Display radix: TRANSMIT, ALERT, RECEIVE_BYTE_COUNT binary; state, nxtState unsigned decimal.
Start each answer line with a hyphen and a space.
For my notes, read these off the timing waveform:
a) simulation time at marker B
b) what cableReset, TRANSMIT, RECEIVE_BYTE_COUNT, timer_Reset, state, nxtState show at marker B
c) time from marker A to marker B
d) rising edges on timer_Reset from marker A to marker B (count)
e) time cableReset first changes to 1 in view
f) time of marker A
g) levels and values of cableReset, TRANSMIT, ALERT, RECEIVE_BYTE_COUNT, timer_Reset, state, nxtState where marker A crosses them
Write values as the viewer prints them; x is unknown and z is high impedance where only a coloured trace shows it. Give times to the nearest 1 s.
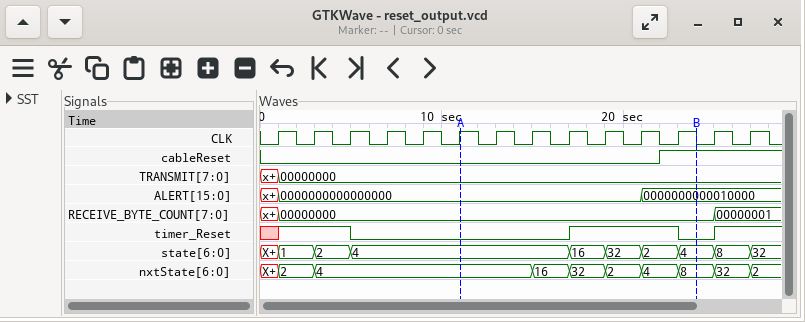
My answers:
- 24 s
- cableReset=1, TRANSMIT=00000000, RECEIVE_BYTE_COUNT=00000000, timer_Reset=0, state=4, nxtState=8
- 13 s
- 1
- 22 s
- 11 s
- cableReset=0, TRANSMIT=00000000, ALERT=0000000000000000, RECEIVE_BYTE_COUNT=00000000, timer_Reset=0, state=4, nxtState=4
